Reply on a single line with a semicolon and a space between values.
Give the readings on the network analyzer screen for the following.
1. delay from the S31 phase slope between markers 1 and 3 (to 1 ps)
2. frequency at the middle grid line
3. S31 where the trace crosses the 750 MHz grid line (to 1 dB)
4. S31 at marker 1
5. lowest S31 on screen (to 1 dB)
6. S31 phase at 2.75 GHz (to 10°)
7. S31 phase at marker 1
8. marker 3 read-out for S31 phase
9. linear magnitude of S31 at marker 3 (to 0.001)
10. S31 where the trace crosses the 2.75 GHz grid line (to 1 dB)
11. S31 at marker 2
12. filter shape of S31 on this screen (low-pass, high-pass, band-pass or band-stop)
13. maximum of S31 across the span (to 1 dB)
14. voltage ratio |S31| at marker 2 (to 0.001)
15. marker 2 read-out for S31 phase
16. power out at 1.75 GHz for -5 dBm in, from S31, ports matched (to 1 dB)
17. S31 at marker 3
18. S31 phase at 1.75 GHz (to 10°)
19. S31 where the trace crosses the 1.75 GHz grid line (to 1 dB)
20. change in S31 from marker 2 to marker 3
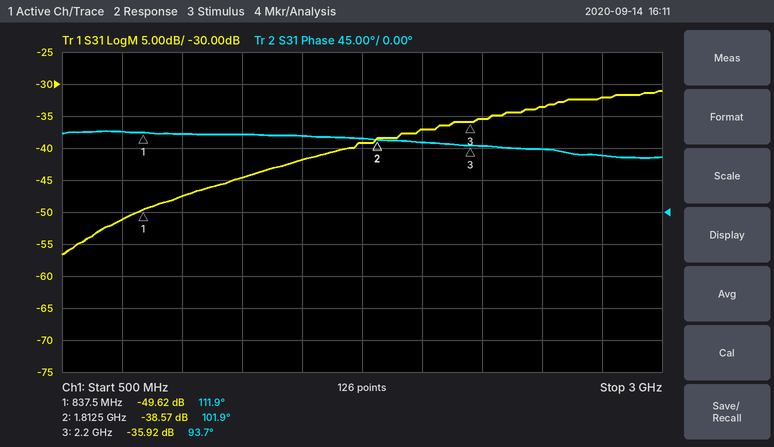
37 ps; 1.75 GHz; -51 dB; -49.62 dB; -57 dB; 80°; 111.9°; 93.7°; 0.016; -32 dB; -38.57 dB; high-pass; -31 dB; 0.012; 101.9°; -44 dBm; -35.92 dB; 100°; -39 dB; 2.65 dB
